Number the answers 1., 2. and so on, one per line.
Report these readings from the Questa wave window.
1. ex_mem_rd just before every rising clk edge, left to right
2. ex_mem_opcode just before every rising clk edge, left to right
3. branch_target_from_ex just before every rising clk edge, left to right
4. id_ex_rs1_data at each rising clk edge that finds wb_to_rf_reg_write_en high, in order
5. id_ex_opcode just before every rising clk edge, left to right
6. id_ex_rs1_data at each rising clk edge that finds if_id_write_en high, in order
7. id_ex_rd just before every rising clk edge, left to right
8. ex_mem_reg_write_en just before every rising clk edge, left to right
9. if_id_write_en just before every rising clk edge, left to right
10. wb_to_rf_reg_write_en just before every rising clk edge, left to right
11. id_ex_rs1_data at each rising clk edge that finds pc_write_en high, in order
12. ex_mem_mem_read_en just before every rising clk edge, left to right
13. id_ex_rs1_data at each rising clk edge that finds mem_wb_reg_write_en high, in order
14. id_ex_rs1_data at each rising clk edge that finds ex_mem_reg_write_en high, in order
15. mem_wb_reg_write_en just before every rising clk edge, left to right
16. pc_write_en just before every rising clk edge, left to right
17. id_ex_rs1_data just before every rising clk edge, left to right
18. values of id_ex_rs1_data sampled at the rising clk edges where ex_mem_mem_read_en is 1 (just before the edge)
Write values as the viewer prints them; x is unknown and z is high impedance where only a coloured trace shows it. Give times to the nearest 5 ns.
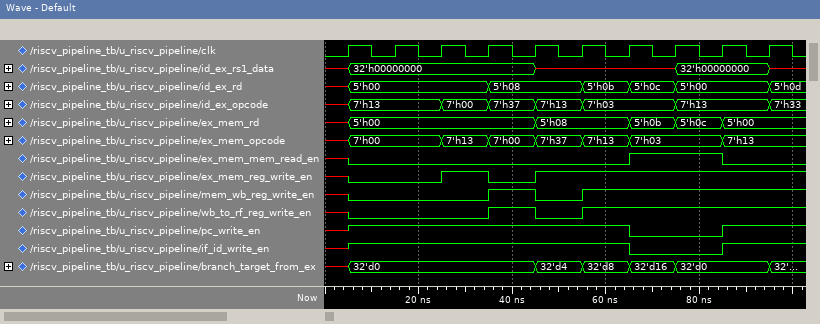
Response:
1. x, 5'h00, 5'h00, 5'h00, 5'h00, 5'h08, 5'h08, 5'h0b, 5'h0c, 5'h00
2. x, 7'h00, 7'h00, 7'h13, 7'h00, 7'h37, 7'h13, 7'h03, 7'h03, 7'h13
3. x, 32'd0, 32'd0, 32'd0, 32'd0, 32'd4, 32'd8, 32'd16, 32'd0, 32'd0
4. 32'h00000000, x, x, 32'h00000000, 32'h00000000
5. x, 7'h13, 7'h13, 7'h00, 7'h37, 7'h13, 7'h03, 7'h03, 7'h13, 7'h13
6. 32'h00000000, 32'h00000000, 32'h00000000, 32'h00000000, x, x, 32'h00000000
7. x, 5'h00, 5'h00, 5'h00, 5'h08, 5'h08, 5'h0b, 5'h0c, 5'h00, 5'h00
8. x 0 0 1 0 1 1 1 1 1
9. x 1 1 1 1 1 1 0 0 1
10. x 0 0 0 1 0 1 1 1 1
11. 32'h00000000, 32'h00000000, 32'h00000000, 32'h00000000, x, x, 32'h00000000
12. x 0 0 0 0 0 0 1 1 0
13. 32'h00000000, x, x, 32'h00000000, 32'h00000000
14. 32'h00000000, x, x, x, 32'h00000000, 32'h00000000
15. x 0 0 0 1 0 1 1 1 1
16. x 1 1 1 1 1 1 0 0 1
17. x, 32'h00000000, 32'h00000000, 32'h00000000, 32'h00000000, x, x, x, 32'h00000000, 32'h00000000
18. x, 32'h00000000
